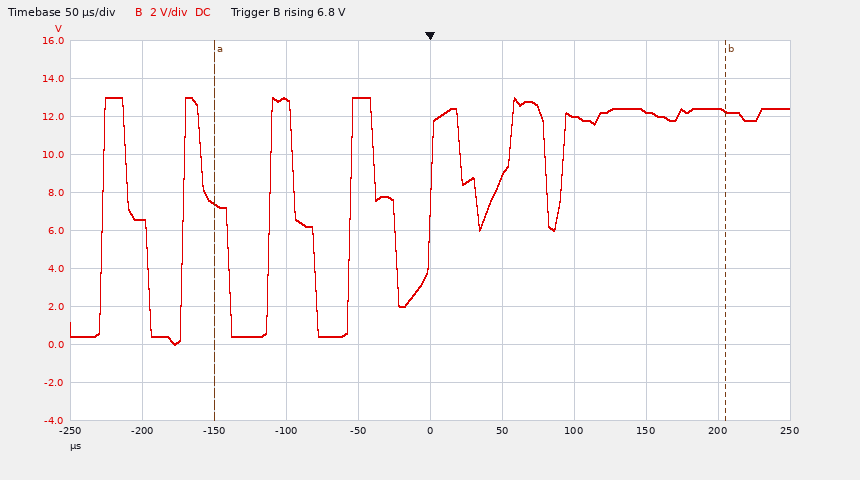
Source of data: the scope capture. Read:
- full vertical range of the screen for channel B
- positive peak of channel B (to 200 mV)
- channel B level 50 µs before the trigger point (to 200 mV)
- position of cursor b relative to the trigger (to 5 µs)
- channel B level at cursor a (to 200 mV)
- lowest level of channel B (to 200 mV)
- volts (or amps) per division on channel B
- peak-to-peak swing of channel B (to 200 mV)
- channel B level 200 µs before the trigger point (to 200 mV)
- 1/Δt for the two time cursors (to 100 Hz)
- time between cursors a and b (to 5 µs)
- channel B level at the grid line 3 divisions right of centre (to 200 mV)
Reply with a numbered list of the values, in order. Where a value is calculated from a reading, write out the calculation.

1. 20 V
2. 13.0 V
3. 13.0 V
4. +205 µs
5. 7.4 V
6. 0.0 V
7. 2 V
8. 13.0 V − (0.0 V) = 13.0 V
9. 6.6 V
10. 1 / 355 µs ≈ 2.8 kHz
11. 355 µs
12. 12.2 V
